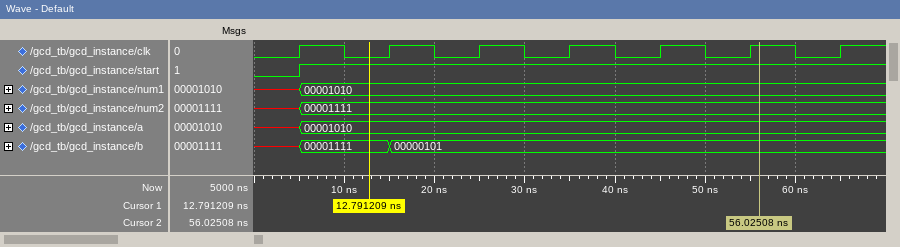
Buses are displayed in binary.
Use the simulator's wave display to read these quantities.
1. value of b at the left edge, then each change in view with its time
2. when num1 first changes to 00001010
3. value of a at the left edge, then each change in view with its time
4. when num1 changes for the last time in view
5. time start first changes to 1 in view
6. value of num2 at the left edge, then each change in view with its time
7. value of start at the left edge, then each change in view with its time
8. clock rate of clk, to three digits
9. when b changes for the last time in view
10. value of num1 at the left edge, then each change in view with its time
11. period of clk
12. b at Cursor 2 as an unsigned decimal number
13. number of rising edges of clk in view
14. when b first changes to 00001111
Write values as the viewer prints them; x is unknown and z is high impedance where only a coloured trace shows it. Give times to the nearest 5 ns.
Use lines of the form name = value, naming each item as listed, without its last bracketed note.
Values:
value of b at the left edge, then each change in view with its time = x, 00001111 at 5 ns, 00000101 at 15 ns
when num1 first changes to 00001010 = 5 ns
value of a at the left edge, then each change in view with its time = x, 00001010 at 5 ns
when num1 changes for the last time in view = 5 ns
time start first changes to 1 in view = 5 ns
value of num2 at the left edge, then each change in view with its time = x, 00001111 at 5 ns
value of start at the left edge, then each change in view with its time = 0, 1 at 5 ns
clock rate of clk, to three digits = 100 MHz
when b changes for the last time in view = 15 ns
value of num1 at the left edge, then each change in view with its time = x, 00001010 at 5 ns
period of clk = 10 ns
b at Cursor 2 as an unsigned decimal number = 5
number of rising edges of clk in view = 7
when b first changes to 00001111 = 5 ns
